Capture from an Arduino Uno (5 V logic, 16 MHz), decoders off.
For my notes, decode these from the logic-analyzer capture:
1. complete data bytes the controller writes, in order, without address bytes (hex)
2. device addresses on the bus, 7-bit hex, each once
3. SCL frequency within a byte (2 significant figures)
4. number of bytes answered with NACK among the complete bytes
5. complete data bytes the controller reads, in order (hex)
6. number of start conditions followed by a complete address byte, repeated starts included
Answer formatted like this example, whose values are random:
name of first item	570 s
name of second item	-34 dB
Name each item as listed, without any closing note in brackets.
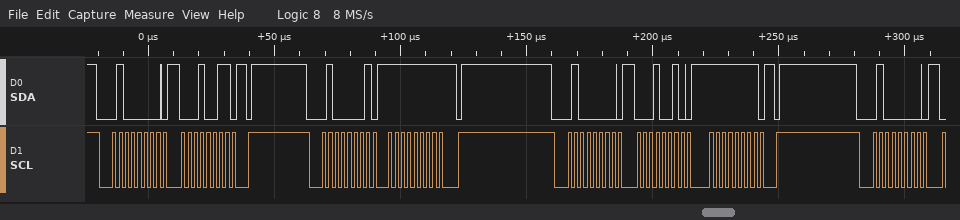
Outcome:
complete data bytes the controller writes, in order, without address bytes	13 12 FF
device addresses on the bus, 7-bit hex, each once	0x20
SCL frequency within a byte	400 kHz
number of bytes answered with NACK among the complete bytes	1
complete data bytes the controller reads, in order	FF
number of start conditions followed by a complete address byte, repeated starts included	4
